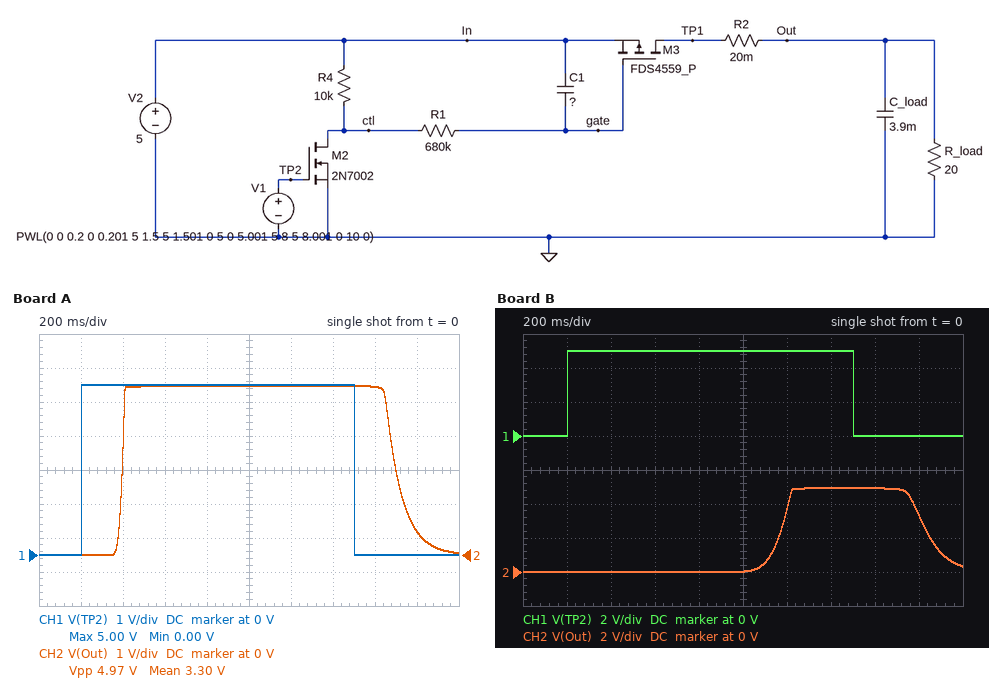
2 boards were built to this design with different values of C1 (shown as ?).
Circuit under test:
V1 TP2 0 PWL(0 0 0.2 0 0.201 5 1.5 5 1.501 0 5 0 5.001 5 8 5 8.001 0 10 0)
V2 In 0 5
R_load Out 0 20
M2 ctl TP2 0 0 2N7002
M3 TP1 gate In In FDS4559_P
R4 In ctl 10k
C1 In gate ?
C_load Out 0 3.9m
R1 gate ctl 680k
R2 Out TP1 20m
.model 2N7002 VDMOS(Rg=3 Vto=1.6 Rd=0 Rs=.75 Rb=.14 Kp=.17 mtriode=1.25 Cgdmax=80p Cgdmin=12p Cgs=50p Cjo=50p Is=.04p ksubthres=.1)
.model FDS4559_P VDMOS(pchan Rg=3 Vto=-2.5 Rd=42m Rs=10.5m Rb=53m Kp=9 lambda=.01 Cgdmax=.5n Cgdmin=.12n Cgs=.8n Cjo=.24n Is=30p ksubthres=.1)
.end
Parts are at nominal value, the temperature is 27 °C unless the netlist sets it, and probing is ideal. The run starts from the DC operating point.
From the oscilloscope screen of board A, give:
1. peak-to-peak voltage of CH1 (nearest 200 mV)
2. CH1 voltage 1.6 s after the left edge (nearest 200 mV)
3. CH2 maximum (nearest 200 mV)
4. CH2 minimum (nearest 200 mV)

5.0 V
0 V
5.0 V
0 V
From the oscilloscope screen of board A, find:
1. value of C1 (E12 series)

330 nF
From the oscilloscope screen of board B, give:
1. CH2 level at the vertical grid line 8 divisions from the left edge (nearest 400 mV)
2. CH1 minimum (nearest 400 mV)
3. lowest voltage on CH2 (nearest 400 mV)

4.8 V
0 V
0 V
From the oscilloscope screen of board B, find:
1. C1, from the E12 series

1.8 µF
